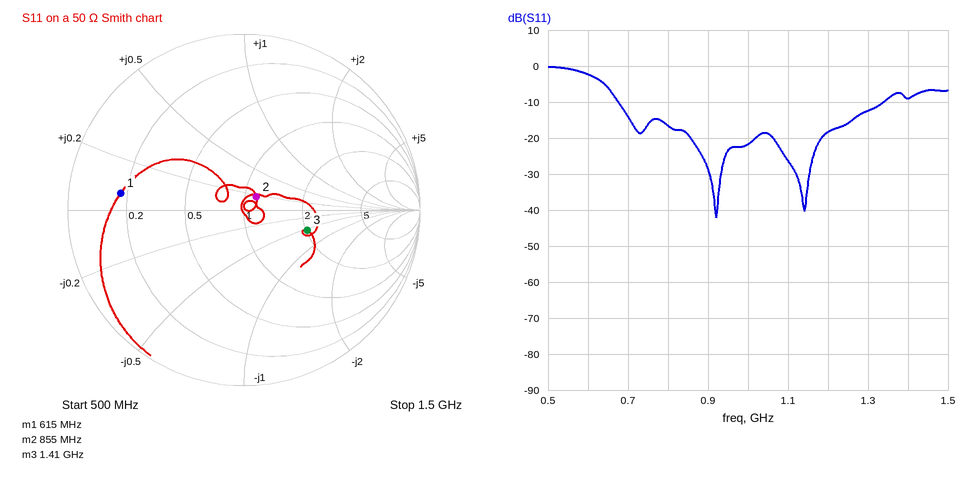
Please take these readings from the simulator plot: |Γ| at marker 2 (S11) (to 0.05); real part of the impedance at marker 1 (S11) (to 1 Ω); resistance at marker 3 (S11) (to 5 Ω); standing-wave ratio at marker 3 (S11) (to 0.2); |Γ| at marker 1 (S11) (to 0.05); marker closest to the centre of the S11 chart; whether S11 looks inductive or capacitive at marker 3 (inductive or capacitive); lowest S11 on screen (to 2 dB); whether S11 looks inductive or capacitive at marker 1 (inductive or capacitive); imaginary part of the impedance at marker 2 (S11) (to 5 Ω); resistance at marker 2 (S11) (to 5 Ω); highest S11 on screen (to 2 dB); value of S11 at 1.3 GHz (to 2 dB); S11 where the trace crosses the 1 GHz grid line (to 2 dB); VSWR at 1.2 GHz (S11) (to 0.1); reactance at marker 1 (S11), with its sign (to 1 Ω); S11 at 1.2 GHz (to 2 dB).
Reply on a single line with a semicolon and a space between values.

0.10; 9 Ω; 100 Ω; 2.2; 0.70; marker 2; capacitive; -42 dB; inductive; +10 Ω; 55 Ω; 0 dB; -12 dB; -22 dB; 1.3; +3 Ω; -18 dB
